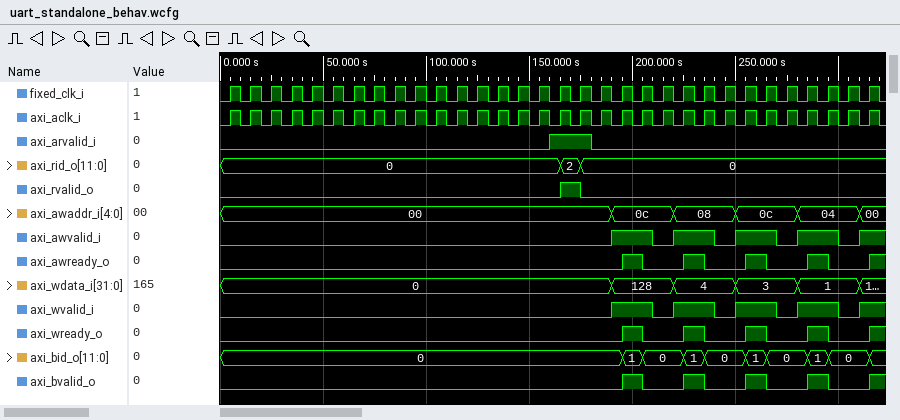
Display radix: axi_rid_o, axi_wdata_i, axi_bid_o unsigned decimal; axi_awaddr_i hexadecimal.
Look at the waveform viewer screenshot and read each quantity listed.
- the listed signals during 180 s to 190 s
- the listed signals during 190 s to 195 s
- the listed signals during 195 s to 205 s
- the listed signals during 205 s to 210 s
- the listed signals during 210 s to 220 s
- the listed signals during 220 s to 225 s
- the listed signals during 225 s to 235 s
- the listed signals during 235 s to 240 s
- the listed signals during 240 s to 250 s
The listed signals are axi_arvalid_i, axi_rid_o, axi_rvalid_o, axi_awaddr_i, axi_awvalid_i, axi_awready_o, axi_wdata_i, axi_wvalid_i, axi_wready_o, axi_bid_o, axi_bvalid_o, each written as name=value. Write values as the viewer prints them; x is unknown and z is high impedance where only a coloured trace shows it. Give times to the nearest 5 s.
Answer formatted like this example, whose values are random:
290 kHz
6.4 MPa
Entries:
axi_arvalid_i=0, axi_rid_o=0, axi_rvalid_o=0, axi_awaddr_i=00, axi_awvalid_i=0, axi_awready_o=0, axi_wdata_i=0, axi_wvalid_i=0, axi_wready_o=0, axi_bid_o=0, axi_bvalid_o=0
axi_arvalid_i=0, axi_rid_o=0, axi_rvalid_o=0, axi_awaddr_i=0c, axi_awvalid_i=1, axi_awready_o=0, axi_wdata_i=128, axi_wvalid_i=1, axi_wready_o=0, axi_bid_o=0, axi_bvalid_o=0
axi_arvalid_i=0, axi_rid_o=0, axi_rvalid_o=0, axi_awaddr_i=0c, axi_awvalid_i=1, axi_awready_o=1, axi_wdata_i=128, axi_wvalid_i=1, axi_wready_o=1, axi_bid_o=1, axi_bvalid_o=1
axi_arvalid_i=0, axi_rid_o=0, axi_rvalid_o=0, axi_awaddr_i=0c, axi_awvalid_i=1, axi_awready_o=0, axi_wdata_i=128, axi_wvalid_i=1, axi_wready_o=0, axi_bid_o=0, axi_bvalid_o=0
axi_arvalid_i=0, axi_rid_o=0, axi_rvalid_o=0, axi_awaddr_i=0c, axi_awvalid_i=0, axi_awready_o=0, axi_wdata_i=128, axi_wvalid_i=0, axi_wready_o=0, axi_bid_o=0, axi_bvalid_o=0
axi_arvalid_i=0, axi_rid_o=0, axi_rvalid_o=0, axi_awaddr_i=08, axi_awvalid_i=1, axi_awready_o=0, axi_wdata_i=4, axi_wvalid_i=1, axi_wready_o=0, axi_bid_o=0, axi_bvalid_o=0
axi_arvalid_i=0, axi_rid_o=0, axi_rvalid_o=0, axi_awaddr_i=08, axi_awvalid_i=1, axi_awready_o=1, axi_wdata_i=4, axi_wvalid_i=1, axi_wready_o=1, axi_bid_o=1, axi_bvalid_o=1
axi_arvalid_i=0, axi_rid_o=0, axi_rvalid_o=0, axi_awaddr_i=08, axi_awvalid_i=1, axi_awready_o=0, axi_wdata_i=4, axi_wvalid_i=1, axi_wready_o=0, axi_bid_o=0, axi_bvalid_o=0
axi_arvalid_i=0, axi_rid_o=0, axi_rvalid_o=0, axi_awaddr_i=08, axi_awvalid_i=0, axi_awready_o=0, axi_wdata_i=4, axi_wvalid_i=0, axi_wready_o=0, axi_bid_o=0, axi_bvalid_o=0
